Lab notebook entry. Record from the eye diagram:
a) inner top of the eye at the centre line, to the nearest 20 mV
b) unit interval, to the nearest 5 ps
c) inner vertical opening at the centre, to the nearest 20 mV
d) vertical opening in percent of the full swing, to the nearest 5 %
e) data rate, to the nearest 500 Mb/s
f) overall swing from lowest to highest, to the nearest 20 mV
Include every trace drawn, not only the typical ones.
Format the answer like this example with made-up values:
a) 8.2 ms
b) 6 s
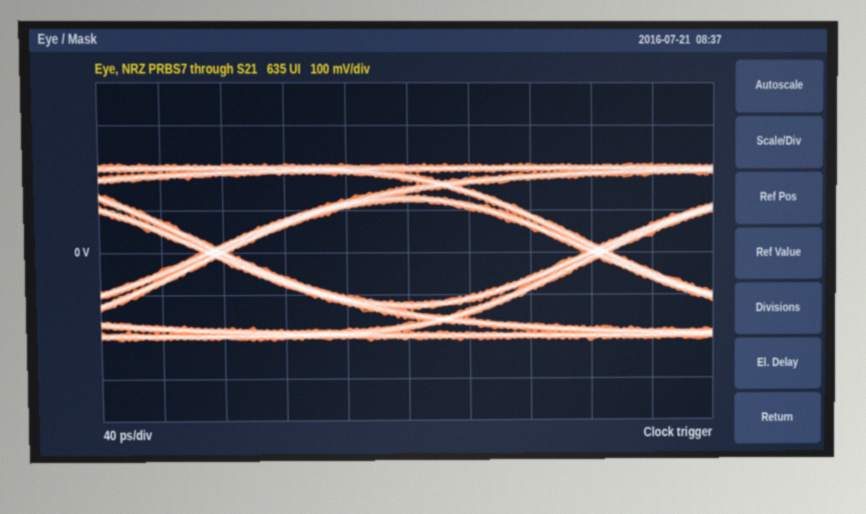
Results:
a) 120 mV
b) 250 ps
c) 240 mV
d) 55 %
e) 4.0 Gb/s
f) 420 mV
